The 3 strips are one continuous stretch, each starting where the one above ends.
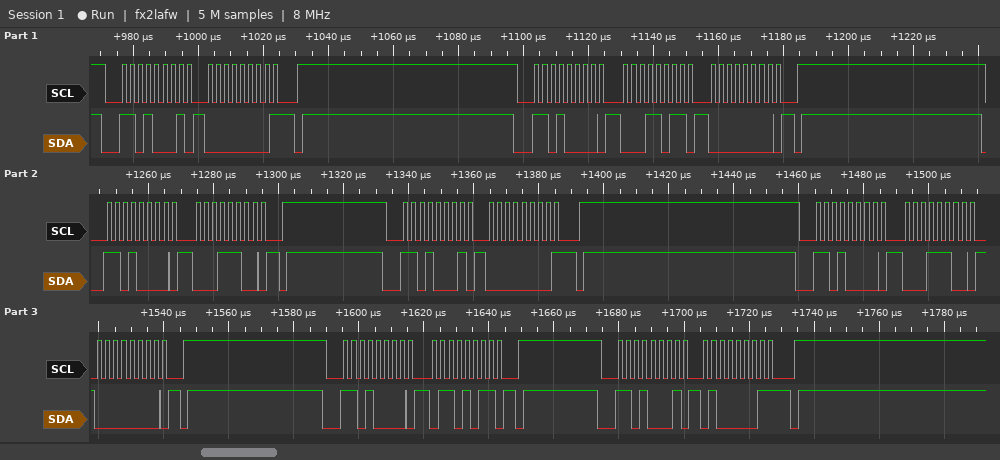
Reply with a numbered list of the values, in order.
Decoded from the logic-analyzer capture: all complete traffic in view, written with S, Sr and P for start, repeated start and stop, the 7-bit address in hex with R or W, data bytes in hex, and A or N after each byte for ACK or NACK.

1. S 68R A 00 N P S 68W A 1B A 00 A P S 68W A 1C A P S 68R A 00 N P S 68W A 1C A 00 A P S 68W A 6B A P S 68R A 41 N P
